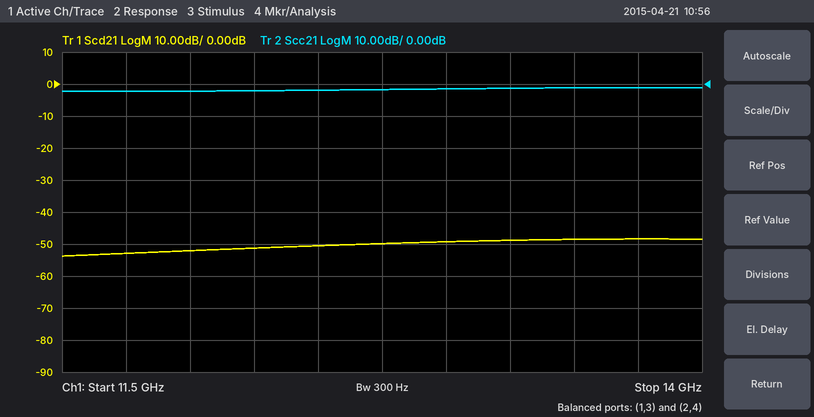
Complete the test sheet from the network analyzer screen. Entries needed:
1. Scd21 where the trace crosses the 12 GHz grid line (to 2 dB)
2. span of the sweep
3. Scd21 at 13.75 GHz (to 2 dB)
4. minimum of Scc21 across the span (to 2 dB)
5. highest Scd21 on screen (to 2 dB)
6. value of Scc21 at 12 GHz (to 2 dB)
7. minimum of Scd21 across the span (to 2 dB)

-52 dB
2.5 GHz
-48 dB
-2 dB
-48 dB
-2 dB
-54 dB
